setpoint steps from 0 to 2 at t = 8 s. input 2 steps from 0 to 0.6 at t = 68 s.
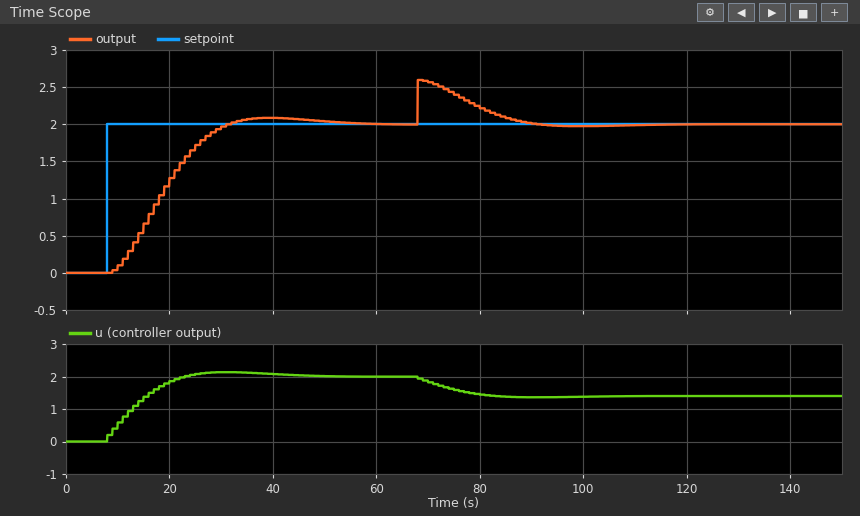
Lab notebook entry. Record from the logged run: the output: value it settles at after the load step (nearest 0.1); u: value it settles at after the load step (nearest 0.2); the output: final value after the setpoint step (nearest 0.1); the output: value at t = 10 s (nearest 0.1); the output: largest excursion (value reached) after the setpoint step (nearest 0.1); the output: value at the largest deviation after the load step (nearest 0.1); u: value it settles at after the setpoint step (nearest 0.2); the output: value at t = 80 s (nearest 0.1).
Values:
2.0
1.4
2.0
0.1
2.1
2.6
2.0
2.2
